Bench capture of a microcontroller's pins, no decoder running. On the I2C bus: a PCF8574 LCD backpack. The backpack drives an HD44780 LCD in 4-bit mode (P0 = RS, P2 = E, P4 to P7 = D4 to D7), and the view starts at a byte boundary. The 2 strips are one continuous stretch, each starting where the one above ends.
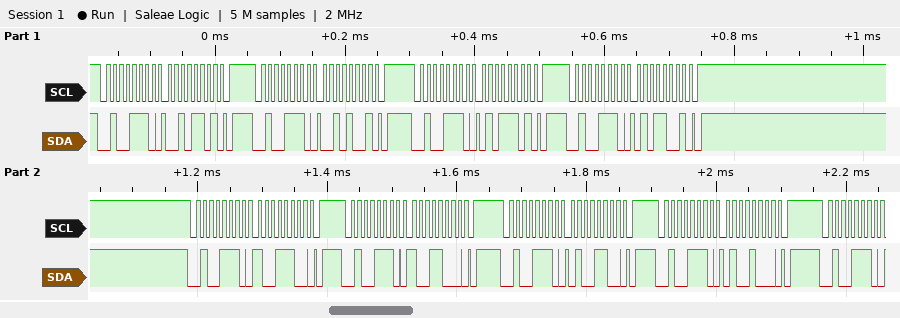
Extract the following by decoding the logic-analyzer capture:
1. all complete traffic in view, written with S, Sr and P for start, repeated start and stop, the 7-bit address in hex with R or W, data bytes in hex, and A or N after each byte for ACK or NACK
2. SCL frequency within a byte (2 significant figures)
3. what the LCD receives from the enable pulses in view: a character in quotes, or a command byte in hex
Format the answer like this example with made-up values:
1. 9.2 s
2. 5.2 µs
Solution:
1. S 27W A 2D A P S 27W A 29 A P S 27W A 5D A P S 27W A 59 A P S 27W A 9C A P S 27W A 98 A P S 27W A 4C A P S 27W A 48 A P S 27W A
2. 100 kHz
3. '%' 0x94
